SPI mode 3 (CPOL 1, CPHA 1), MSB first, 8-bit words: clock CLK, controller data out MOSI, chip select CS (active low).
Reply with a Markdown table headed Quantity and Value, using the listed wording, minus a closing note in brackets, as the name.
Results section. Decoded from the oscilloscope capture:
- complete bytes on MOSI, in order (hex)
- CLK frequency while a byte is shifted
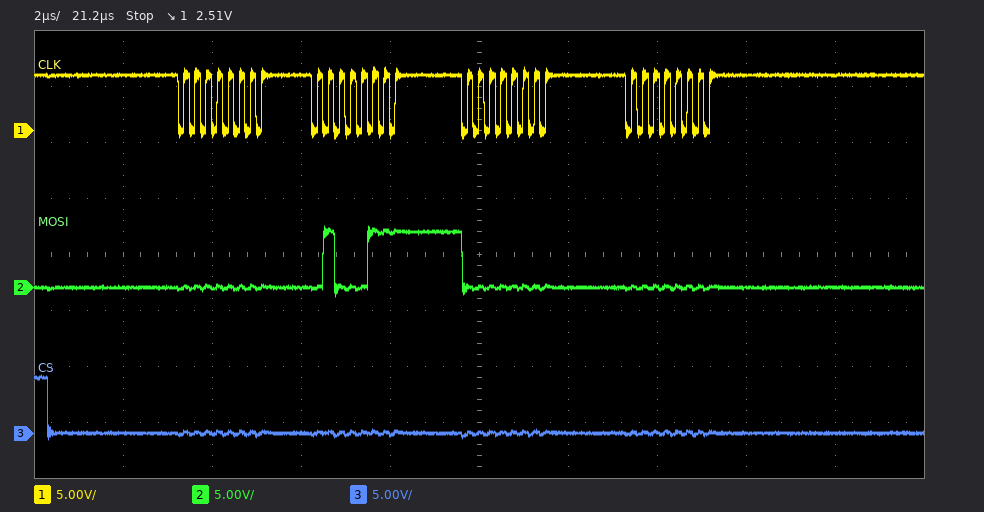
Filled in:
| Quantity | Value |
|---|---|
| complete bytes on MOSI, in order | 00 47 00 00 |
| CLK frequency while a byte is shifted | 4 MHz |
